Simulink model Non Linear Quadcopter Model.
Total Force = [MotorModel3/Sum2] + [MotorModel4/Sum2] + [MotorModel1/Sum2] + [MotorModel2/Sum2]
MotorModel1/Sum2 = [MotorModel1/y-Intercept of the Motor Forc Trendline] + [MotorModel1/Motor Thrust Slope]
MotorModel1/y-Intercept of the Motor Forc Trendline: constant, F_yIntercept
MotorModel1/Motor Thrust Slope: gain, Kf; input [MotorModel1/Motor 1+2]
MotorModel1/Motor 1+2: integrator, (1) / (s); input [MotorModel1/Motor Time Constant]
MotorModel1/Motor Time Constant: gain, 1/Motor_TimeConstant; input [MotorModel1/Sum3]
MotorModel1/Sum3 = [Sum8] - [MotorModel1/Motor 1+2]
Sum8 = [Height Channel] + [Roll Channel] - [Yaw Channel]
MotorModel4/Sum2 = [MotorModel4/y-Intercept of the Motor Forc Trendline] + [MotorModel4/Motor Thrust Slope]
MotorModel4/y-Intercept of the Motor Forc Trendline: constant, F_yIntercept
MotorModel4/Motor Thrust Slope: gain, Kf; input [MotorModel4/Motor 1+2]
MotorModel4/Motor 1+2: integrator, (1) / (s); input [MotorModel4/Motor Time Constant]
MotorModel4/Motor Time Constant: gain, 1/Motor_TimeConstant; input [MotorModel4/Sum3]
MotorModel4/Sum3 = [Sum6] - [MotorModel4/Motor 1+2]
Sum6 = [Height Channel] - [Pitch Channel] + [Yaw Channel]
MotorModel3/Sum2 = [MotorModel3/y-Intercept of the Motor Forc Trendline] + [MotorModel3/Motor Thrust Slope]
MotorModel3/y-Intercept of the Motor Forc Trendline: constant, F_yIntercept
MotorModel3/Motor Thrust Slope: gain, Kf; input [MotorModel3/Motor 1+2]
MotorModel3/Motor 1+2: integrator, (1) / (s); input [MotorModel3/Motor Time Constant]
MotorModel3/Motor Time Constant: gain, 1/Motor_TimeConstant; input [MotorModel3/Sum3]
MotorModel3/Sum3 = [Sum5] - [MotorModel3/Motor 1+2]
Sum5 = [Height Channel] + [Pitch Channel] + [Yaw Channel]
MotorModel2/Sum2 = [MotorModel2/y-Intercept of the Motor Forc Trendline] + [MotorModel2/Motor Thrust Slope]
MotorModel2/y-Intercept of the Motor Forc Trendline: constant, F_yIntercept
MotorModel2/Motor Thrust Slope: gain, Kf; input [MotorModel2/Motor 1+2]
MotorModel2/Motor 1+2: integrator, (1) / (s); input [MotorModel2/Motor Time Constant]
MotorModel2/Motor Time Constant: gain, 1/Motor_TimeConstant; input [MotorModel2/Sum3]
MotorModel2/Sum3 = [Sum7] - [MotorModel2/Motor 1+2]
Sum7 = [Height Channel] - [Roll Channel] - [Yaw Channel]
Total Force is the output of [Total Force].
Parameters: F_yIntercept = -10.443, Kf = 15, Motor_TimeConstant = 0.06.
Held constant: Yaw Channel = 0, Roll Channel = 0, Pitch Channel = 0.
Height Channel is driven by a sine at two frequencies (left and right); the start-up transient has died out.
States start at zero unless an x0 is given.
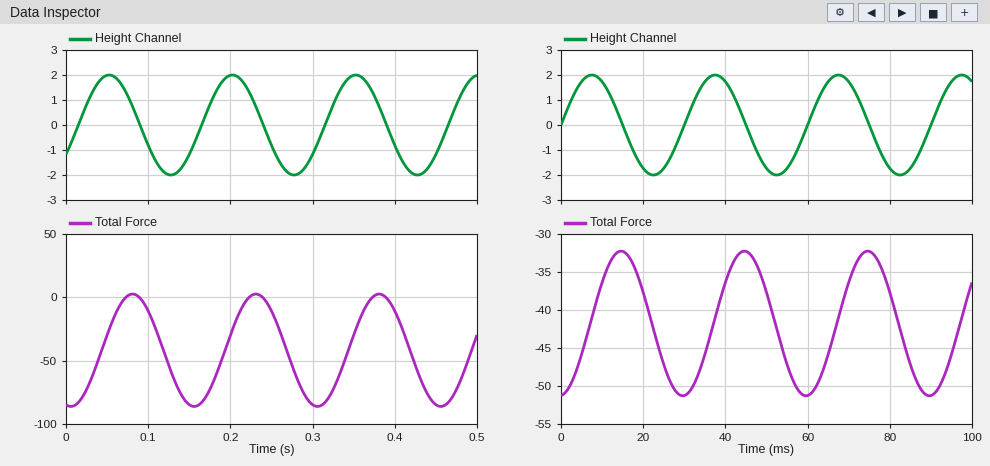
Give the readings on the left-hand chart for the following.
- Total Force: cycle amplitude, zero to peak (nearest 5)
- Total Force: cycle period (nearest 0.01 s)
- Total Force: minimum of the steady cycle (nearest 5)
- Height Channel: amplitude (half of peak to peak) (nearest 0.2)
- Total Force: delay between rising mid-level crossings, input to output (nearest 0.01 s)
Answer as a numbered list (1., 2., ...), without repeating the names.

1. 45
2. 0.15 s
3. -85
4. 2.0
5. 0.03 s
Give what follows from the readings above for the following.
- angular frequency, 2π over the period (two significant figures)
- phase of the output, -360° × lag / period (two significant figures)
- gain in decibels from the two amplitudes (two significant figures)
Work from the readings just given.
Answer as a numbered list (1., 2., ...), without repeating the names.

1. 42 rad/s
2. -72°
3. 27 dB
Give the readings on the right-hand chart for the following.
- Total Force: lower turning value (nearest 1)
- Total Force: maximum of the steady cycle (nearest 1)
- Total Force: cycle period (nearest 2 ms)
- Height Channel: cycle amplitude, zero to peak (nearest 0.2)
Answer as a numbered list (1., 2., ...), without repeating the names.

1. -51
2. -32
3. 30 ms
4. 2.0
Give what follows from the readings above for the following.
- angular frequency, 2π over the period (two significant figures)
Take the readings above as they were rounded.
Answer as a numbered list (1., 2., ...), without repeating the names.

1. 0.21 rad/ms
